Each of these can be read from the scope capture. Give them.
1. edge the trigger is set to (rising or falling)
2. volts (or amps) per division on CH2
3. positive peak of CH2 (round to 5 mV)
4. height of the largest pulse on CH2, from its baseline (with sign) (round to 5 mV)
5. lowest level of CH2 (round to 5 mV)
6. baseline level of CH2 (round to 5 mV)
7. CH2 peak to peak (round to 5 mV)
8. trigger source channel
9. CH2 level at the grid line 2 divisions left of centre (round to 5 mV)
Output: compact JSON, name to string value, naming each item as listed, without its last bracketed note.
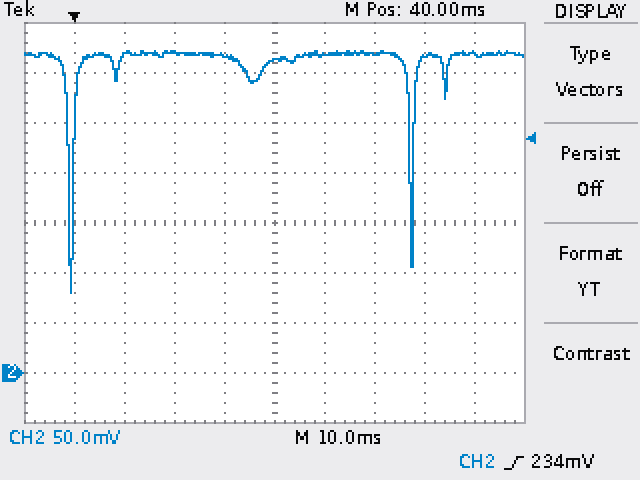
{"edge the trigger is set to": "rising", "volts (or amps) per division on CH2": "50 mV", "positive peak of CH2": "320 mV", "height of the largest pulse on CH2, from its baseline (with sign)": "-240 mV", "lowest level of CH2": "80 mV", "baseline level of CH2": "320 mV", "CH2 peak to peak": "240 mV", "trigger source channel": "CH2", "CH2 level at the grid line 2 divisions left of centre": "320 mV"}
